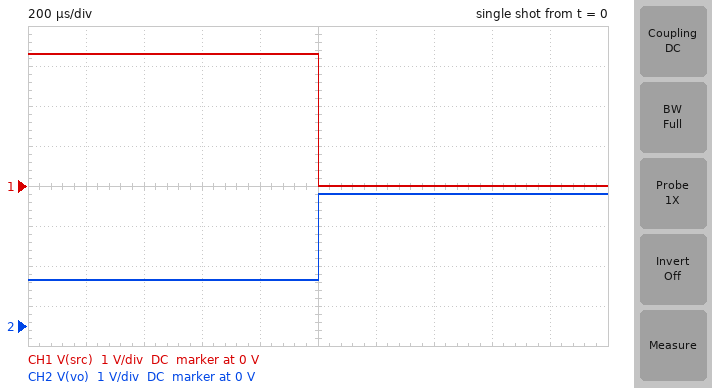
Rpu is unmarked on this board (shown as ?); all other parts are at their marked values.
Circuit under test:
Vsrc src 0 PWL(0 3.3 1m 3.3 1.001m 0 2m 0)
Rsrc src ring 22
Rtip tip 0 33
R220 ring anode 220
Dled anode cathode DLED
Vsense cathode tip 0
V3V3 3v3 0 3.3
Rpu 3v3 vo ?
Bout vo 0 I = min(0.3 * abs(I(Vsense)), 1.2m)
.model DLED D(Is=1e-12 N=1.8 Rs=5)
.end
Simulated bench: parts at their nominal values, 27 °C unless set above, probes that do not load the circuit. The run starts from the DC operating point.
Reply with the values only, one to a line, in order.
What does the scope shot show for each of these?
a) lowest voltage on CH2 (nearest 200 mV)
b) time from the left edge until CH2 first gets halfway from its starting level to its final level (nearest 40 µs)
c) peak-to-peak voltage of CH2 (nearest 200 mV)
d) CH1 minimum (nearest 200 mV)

1.2 V
1.00 ms
2.2 V
0 V
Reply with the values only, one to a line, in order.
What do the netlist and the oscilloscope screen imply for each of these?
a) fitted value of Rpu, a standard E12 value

1.8 kΩ
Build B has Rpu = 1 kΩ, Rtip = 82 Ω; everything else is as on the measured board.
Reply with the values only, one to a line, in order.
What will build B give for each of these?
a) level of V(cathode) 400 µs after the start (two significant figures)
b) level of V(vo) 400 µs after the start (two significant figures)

560 mV
2.1 V
